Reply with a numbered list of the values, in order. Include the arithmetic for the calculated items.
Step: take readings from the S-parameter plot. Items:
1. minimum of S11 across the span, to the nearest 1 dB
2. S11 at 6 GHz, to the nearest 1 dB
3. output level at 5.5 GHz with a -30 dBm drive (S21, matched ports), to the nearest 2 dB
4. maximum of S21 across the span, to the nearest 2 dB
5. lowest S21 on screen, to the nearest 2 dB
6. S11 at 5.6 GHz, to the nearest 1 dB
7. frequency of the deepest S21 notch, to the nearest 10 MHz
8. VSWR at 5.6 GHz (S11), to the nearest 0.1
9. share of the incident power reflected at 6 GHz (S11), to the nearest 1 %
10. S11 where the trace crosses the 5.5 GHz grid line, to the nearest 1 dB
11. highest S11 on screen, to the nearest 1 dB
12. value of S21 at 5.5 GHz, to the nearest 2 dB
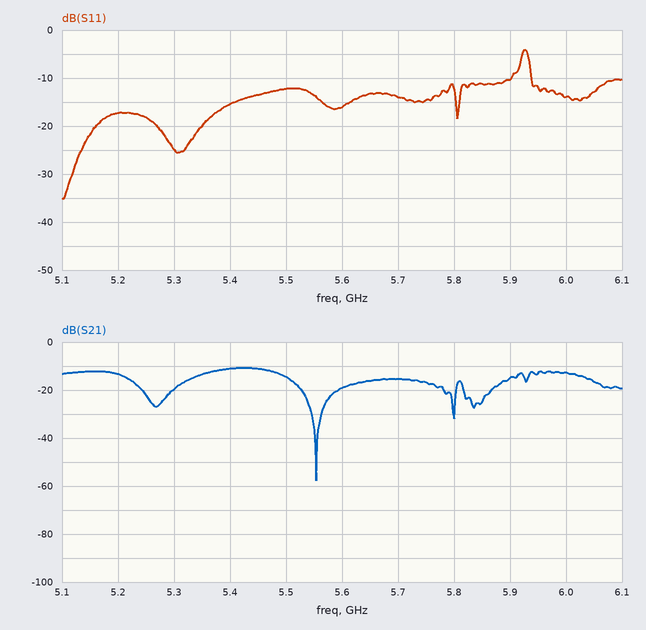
1. -35 dB
2. -14 dB
3. -30 dBm + (-14 dB) = -44 dBm
4. -10 dB
5. -58 dB
6. -16 dB
7. 5.55 GHz
8. |Γ| = 10^(-16/20) = 0.1585; VSWR = (1 + 0.1585)/(1 − 0.1585) ≈ 1.4
9. 10^(-14/10) ≈ 4 %
10. -12 dB
11. -4 dB
12. -14 dB
